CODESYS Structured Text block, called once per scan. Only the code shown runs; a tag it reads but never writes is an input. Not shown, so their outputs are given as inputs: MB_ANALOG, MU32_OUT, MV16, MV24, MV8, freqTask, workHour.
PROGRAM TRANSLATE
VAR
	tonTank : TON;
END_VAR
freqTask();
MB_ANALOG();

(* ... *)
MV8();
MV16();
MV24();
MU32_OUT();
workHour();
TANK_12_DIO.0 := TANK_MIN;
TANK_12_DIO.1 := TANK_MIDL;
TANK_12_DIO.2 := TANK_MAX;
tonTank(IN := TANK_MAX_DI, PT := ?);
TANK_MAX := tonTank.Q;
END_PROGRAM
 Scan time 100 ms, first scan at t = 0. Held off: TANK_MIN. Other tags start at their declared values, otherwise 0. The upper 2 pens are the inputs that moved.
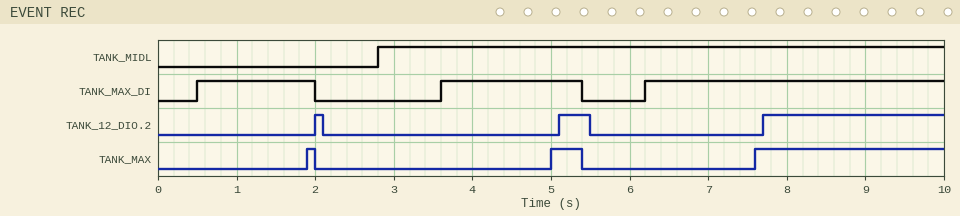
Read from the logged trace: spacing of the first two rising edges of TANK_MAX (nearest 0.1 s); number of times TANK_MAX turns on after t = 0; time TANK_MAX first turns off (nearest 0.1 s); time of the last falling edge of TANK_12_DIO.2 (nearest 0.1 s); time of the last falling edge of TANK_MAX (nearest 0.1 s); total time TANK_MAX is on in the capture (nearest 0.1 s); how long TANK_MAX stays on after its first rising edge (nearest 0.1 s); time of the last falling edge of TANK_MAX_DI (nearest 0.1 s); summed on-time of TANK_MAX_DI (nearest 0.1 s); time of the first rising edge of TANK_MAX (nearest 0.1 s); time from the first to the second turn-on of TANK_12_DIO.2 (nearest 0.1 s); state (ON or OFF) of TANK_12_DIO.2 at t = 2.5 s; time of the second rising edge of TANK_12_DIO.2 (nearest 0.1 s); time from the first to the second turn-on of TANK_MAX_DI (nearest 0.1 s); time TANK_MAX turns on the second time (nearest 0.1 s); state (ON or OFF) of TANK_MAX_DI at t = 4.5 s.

3.1 s
3
2.0 s
5.5 s
5.4 s
2.9 s
0.1 s
5.4 s
7.1 s
1.9 s
3.1 s
OFF
5.1 s
3.1 s
5.0 s
ON
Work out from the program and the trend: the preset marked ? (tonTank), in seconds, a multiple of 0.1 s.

1.4 s
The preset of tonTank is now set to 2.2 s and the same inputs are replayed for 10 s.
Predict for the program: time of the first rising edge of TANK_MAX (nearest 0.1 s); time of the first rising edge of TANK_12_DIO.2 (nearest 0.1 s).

8.4 s
8.5 s
